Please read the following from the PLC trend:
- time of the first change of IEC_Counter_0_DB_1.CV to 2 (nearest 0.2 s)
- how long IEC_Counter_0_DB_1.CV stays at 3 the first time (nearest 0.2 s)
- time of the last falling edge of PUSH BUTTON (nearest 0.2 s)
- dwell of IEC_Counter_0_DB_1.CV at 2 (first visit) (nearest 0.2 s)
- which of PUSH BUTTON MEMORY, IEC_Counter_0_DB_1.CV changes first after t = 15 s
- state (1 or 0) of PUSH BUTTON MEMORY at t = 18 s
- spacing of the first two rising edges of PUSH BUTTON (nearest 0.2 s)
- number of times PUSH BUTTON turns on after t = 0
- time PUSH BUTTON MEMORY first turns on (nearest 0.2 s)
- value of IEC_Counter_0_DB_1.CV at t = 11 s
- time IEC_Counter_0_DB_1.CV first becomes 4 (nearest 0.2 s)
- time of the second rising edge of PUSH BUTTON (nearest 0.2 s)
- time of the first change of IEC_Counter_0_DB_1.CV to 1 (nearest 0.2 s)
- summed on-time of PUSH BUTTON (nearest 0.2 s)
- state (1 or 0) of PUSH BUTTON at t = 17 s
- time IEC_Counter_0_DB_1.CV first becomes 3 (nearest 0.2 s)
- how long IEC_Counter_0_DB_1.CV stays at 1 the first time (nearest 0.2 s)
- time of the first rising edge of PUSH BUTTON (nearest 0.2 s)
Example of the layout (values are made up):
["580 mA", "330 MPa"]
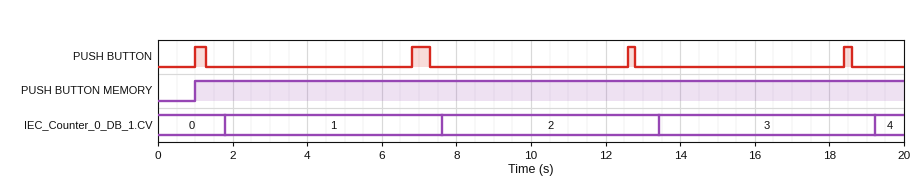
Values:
["7.6 s", "5.8 s", "18.6 s", "5.8 s", "IEC_Counter_0_DB_1.CV", "1", "5.8 s", "4", "1.0 s", "2", "19.2 s", "6.8 s", "1.8 s", "1.2 s", "0", "13.4 s", "5.8 s", "1.0 s"]
